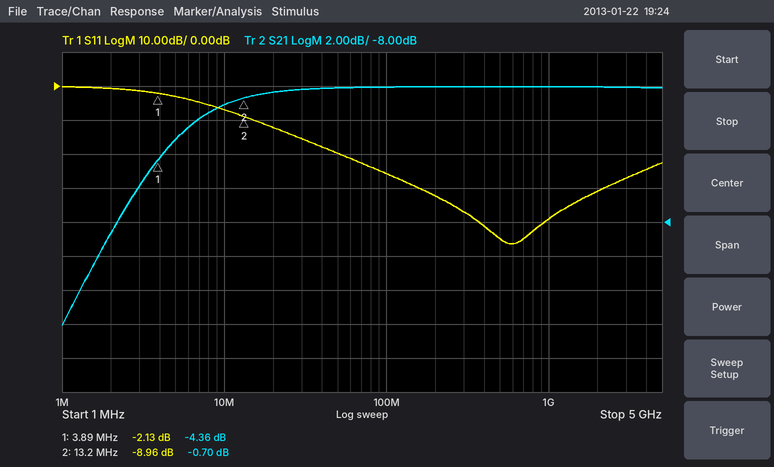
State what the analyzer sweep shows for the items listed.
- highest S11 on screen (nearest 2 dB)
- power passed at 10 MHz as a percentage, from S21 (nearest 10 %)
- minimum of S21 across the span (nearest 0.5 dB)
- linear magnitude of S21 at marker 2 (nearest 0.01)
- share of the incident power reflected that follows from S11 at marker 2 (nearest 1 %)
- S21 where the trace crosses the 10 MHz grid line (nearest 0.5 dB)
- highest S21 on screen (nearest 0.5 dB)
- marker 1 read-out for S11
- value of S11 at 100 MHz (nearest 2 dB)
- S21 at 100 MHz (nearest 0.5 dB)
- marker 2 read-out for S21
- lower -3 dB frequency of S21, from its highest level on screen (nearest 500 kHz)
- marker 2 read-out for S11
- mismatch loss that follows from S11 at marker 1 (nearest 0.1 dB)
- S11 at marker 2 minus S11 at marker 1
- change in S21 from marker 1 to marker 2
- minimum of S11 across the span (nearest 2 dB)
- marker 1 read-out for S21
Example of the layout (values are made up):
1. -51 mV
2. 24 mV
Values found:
1. 0 dB
2. 80 %
3. -14.0 dB
4. 0.92
5. 13 %
6. -1.0 dB
7. 0.0 dB
8. -2.13 dB
9. -26 dB
10. 0.0 dB
11. -0.70 dB
12. 5.0 MHz
13. -8.96 dB
14. 4.1 dB
15. -6.83 dB
16. 3.66 dB
17. -46 dB
18. -4.36 dB
